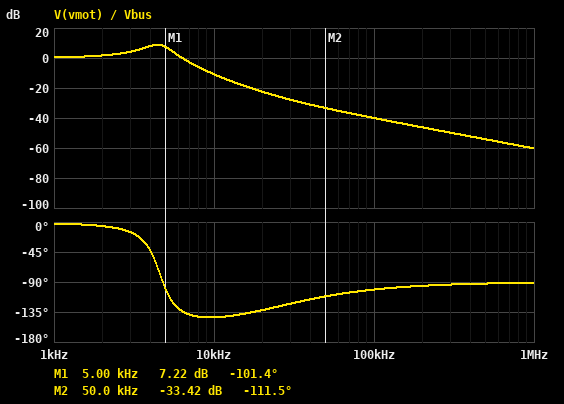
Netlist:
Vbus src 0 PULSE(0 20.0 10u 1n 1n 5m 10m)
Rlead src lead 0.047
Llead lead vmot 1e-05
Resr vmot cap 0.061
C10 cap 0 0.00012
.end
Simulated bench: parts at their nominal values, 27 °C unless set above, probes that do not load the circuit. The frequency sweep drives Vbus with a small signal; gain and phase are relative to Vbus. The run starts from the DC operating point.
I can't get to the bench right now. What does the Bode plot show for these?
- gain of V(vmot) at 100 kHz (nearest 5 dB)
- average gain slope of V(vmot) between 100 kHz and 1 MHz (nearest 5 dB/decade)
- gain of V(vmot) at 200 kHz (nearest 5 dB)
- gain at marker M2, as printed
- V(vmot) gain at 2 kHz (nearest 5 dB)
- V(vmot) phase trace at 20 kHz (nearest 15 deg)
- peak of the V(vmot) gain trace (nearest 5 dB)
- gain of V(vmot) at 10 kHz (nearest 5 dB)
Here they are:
-40 dB
-20 dB/decade
-45 dB
-33.42 dB
0 dB
-135 deg
10 dB
-10 dB
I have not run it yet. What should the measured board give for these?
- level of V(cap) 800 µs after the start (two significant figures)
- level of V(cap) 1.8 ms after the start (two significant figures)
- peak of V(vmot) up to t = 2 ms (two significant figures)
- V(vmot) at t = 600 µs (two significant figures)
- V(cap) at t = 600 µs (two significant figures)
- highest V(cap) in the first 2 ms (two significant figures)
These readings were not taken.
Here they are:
20 V
20 V
31 V
20 V
21 V
31 V
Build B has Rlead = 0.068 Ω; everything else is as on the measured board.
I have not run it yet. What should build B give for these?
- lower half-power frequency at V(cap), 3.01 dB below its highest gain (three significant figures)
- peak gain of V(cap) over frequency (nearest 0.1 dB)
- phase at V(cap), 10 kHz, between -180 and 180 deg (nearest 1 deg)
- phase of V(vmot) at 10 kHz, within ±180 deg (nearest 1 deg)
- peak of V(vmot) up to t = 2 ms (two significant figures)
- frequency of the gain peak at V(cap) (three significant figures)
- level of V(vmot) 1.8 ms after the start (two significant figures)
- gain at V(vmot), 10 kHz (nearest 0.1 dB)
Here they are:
3.13 kHz
7.2 dB
-165 deg
-141 deg
30 V
4.36 kHz
20 V
-10.9 dB
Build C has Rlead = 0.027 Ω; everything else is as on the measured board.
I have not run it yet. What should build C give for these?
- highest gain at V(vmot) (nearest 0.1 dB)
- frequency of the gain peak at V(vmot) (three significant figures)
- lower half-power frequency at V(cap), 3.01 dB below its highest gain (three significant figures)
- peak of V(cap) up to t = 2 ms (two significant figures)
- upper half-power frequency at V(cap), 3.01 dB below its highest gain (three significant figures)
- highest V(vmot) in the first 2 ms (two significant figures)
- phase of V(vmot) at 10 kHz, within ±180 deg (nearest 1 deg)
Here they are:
10.6 dB
4.49 kHz
3.71 kHz
32 V
5.15 kHz
33 V
-145 deg
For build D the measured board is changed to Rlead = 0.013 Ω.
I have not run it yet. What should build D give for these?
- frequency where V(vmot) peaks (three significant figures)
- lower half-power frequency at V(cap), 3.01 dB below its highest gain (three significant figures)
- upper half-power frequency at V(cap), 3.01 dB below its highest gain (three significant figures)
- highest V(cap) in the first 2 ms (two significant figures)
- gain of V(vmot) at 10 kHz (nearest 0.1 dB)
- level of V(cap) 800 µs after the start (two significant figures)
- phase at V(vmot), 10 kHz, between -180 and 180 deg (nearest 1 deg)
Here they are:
4.52 kHz
3.88 kHz
5.08 kHz
33 V
-10.7 dB
21 V
-147 deg
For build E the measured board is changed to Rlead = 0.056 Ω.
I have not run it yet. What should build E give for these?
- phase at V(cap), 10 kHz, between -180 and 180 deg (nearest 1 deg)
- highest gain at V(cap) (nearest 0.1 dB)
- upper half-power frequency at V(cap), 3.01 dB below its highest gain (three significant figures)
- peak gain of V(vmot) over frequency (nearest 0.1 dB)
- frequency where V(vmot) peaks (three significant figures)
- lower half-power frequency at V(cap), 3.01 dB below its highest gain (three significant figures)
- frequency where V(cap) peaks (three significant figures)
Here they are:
-167 deg
8.0 dB
5.27 kHz
8.2 dB
4.41 kHz
3.32 kHz
4.40 kHz
